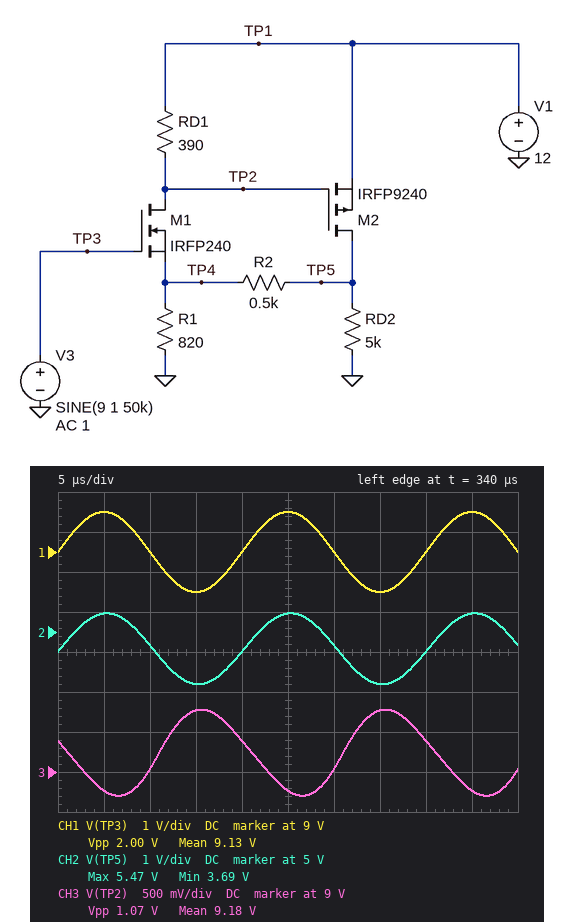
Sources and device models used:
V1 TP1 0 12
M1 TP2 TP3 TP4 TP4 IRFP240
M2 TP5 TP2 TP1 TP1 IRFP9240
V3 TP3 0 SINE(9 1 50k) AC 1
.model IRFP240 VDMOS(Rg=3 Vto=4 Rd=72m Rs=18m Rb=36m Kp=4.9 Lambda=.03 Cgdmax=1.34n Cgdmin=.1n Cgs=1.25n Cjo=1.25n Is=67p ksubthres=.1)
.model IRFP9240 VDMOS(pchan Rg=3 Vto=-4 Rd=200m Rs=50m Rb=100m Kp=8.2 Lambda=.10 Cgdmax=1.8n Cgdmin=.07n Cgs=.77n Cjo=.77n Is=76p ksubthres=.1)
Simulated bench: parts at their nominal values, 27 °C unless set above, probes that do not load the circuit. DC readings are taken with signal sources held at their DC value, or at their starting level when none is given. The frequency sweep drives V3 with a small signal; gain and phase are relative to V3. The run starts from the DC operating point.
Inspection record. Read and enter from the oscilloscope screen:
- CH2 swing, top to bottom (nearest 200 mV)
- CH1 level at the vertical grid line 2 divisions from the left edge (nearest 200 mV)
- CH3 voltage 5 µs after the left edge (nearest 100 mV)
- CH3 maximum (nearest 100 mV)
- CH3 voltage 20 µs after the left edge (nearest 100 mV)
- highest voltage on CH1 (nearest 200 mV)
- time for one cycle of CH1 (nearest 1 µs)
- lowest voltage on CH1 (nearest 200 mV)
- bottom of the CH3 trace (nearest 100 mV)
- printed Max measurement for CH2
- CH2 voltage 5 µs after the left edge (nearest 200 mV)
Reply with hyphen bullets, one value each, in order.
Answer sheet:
- 1.8 V
- 9.0 V
- 8.8 V
- 9.8 V
- 9.4 V
- 10.0 V
- 20 µs
- 8.0 V
- 8.7 V
- 5.47 V
- 5.4 V
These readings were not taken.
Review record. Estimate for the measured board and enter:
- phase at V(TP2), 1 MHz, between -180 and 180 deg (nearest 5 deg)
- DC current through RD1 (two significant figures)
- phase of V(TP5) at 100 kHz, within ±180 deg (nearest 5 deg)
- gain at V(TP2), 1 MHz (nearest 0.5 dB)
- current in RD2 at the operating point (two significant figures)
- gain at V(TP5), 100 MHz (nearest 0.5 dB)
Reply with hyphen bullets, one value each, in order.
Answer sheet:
- 35 deg
- 7.1 mA
- -10 deg
- -6.5 dB
- 920 µA
- -18.0 dB
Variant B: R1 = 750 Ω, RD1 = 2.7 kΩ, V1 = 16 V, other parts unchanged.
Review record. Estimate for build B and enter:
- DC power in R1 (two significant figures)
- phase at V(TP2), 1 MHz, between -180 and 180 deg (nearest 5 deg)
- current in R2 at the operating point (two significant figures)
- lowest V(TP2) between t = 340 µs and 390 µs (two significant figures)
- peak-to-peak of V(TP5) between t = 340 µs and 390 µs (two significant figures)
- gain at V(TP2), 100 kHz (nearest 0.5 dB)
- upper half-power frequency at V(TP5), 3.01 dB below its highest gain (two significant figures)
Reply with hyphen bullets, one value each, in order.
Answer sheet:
- 35 mW
- 150 deg
- 5.4 mA
- 12 V
- 3.3 V
- -34.0 dB
- 5.2 MHz
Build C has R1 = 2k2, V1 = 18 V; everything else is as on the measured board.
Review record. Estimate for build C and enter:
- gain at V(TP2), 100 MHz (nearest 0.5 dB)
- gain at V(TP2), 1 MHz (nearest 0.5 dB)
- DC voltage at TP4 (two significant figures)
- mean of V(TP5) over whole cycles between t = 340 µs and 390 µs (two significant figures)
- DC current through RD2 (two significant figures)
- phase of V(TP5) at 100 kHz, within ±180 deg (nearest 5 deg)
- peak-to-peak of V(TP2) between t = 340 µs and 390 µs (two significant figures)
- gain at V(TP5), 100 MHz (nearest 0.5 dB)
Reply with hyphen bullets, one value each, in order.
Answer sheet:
- -7.5 dB
- -12.0 dB
- 5.1 V
- 4.6 V
- 930 µA
- -5 deg
- 490 mV
- -20.5 dB
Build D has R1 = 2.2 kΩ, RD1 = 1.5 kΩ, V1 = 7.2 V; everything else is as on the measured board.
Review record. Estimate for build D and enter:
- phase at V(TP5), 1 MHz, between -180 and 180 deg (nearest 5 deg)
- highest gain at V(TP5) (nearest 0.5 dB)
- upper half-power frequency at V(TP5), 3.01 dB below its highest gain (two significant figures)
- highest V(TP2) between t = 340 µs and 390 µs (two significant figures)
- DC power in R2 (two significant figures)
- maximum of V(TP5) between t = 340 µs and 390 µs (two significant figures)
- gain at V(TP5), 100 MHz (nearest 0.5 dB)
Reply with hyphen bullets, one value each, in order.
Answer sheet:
- 0 deg
- -5.0 dB
- 31 MHz
- 4.2 V
- 220 µW
- 3.8 V
- -15.0 dB
